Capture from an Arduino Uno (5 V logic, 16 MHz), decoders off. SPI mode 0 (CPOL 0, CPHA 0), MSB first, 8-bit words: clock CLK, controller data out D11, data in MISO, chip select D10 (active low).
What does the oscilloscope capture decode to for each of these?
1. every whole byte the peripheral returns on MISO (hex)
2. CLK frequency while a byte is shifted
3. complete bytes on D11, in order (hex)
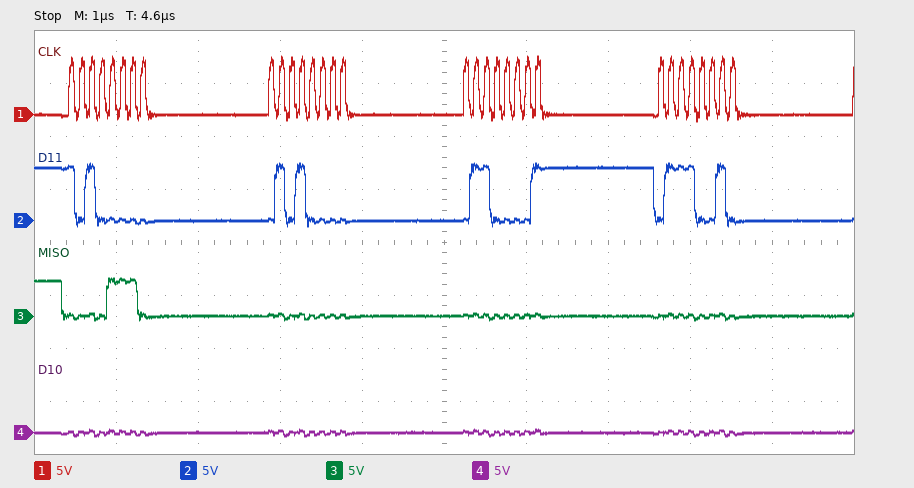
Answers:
0E 00 00 00
8 MHz
A0 50 61 72
